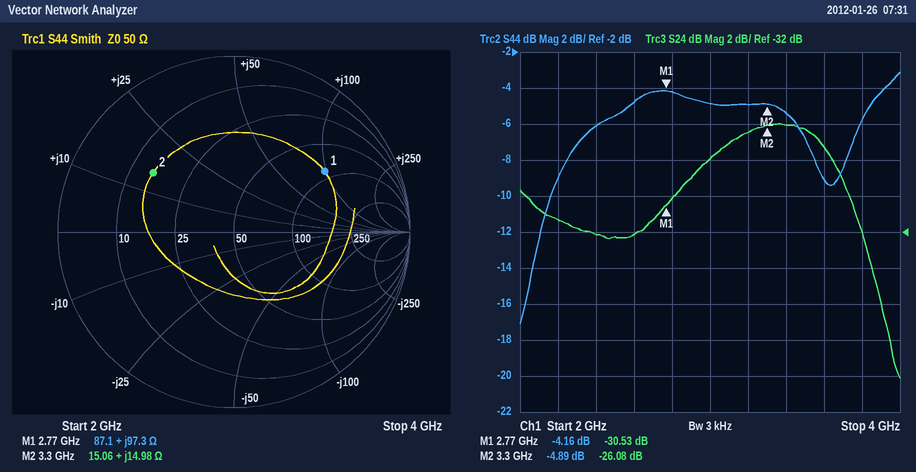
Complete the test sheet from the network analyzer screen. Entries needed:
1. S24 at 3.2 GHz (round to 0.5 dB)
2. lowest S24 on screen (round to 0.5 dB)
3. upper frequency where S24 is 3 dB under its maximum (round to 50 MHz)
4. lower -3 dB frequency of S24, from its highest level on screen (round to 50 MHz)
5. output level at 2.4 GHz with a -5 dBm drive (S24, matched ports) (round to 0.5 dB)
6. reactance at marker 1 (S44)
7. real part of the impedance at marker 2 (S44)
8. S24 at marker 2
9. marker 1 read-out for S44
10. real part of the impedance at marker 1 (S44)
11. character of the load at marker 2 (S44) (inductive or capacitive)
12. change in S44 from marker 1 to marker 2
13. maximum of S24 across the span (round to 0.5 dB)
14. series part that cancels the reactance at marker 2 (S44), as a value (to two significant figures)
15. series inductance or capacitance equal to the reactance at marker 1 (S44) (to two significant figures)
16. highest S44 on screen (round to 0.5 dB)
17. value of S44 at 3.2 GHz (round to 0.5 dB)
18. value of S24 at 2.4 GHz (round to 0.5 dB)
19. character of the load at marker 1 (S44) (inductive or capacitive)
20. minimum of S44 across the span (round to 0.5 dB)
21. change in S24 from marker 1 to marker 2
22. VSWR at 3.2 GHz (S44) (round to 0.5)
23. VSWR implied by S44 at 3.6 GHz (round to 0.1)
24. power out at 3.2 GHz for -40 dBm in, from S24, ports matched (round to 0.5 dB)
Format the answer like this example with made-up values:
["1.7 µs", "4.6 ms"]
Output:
["-26.5 dB", "-40.0 dB", "3.70 GHz", "2.90 GHz", "-37.0 dBm", "+97.3 Ω", "15.06 Ω", "-26.08 dB", "-4.16 dB", "87.1 Ω", "inductive", "-0.73 dB", "-26.0 dB", "3.2 pF", "5.6 nH", "-3.0 dB", "-5.0 dB", "-32.0 dB", "inductive", "-17.0 dB", "4.45 dB", "3.5", "2.1", "-66.5 dBm"]
